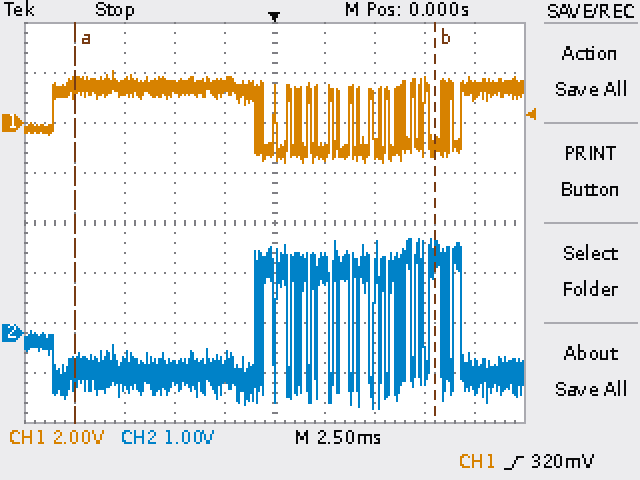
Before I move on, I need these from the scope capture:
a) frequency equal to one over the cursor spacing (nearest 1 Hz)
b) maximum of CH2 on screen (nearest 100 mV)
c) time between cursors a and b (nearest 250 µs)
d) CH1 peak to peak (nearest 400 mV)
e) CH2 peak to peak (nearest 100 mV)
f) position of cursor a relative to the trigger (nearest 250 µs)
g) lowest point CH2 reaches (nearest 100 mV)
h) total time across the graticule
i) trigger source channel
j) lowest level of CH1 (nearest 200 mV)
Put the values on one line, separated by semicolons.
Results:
56 Hz; 1.9 V; 18.00 ms; 3.6 V; 3.4 V; -10.00 ms; -1.5 V; 25 ms; CH1; -1.6 V
